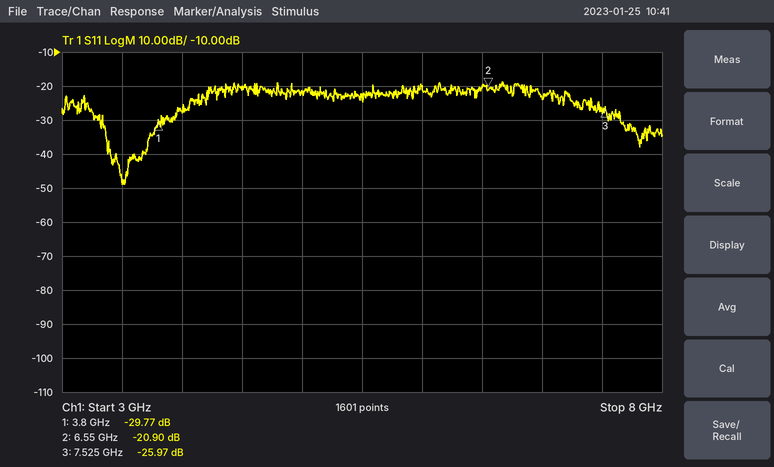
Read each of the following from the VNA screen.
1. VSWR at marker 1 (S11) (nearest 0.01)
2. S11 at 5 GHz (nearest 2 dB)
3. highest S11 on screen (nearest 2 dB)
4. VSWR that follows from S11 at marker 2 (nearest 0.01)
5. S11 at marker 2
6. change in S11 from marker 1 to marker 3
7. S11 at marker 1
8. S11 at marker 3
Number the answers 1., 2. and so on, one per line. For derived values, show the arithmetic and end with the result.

1. (1 + 0.0325)/(1 − 0.0325) ≈ 1.07
2. -22 dB
3. -18 dB
4. (1 + 0.0902)/(1 − 0.0902) ≈ 1.20
5. -20.90 dB
6. -25.97 − (-29.77) = 3.80 dB
7. -29.77 dB
8. -25.97 dB
